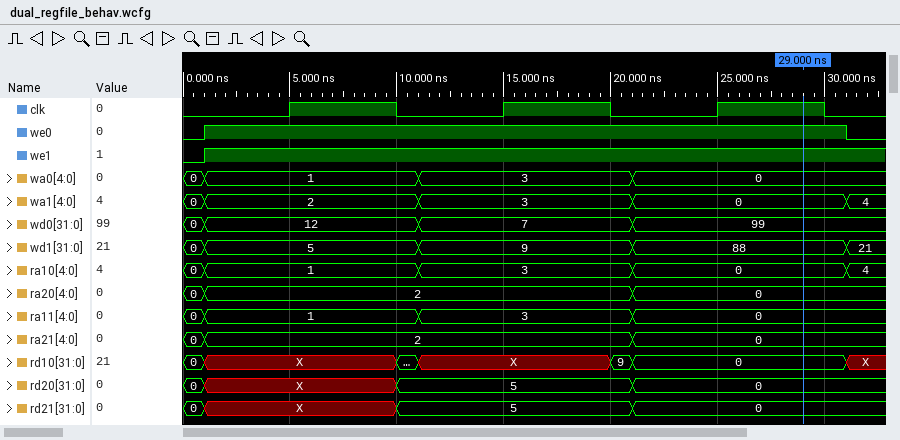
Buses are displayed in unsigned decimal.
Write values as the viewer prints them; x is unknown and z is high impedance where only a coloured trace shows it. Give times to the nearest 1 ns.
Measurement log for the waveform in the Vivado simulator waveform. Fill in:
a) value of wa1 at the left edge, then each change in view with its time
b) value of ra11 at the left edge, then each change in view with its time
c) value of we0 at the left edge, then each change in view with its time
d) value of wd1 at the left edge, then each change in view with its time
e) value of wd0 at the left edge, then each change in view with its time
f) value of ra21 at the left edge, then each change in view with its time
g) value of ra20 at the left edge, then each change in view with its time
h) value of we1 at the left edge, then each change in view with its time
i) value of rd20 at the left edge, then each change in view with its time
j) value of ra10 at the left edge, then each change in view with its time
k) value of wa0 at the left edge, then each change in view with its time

0, 2 at 1 ns, 3 at 11 ns, 0 at 21 ns, 4 at 31 ns
0, 1 at 1 ns, 3 at 11 ns, 0 at 21 ns
0, 1 at 1 ns, 0 at 31 ns
0, 5 at 1 ns, 9 at 11 ns, 88 at 21 ns, 21 at 31 ns
0, 12 at 1 ns, 7 at 11 ns, 99 at 21 ns
0, 2 at 1 ns, 0 at 21 ns
0, 2 at 1 ns, 0 at 21 ns
0, 1 at 1 ns
0, X at 1 ns, 5 at 10 ns, 0 at 21 ns
0, 1 at 1 ns, 3 at 11 ns, 0 at 21 ns, 4 at 31 ns
0, 1 at 1 ns, 3 at 11 ns, 0 at 21 ns
